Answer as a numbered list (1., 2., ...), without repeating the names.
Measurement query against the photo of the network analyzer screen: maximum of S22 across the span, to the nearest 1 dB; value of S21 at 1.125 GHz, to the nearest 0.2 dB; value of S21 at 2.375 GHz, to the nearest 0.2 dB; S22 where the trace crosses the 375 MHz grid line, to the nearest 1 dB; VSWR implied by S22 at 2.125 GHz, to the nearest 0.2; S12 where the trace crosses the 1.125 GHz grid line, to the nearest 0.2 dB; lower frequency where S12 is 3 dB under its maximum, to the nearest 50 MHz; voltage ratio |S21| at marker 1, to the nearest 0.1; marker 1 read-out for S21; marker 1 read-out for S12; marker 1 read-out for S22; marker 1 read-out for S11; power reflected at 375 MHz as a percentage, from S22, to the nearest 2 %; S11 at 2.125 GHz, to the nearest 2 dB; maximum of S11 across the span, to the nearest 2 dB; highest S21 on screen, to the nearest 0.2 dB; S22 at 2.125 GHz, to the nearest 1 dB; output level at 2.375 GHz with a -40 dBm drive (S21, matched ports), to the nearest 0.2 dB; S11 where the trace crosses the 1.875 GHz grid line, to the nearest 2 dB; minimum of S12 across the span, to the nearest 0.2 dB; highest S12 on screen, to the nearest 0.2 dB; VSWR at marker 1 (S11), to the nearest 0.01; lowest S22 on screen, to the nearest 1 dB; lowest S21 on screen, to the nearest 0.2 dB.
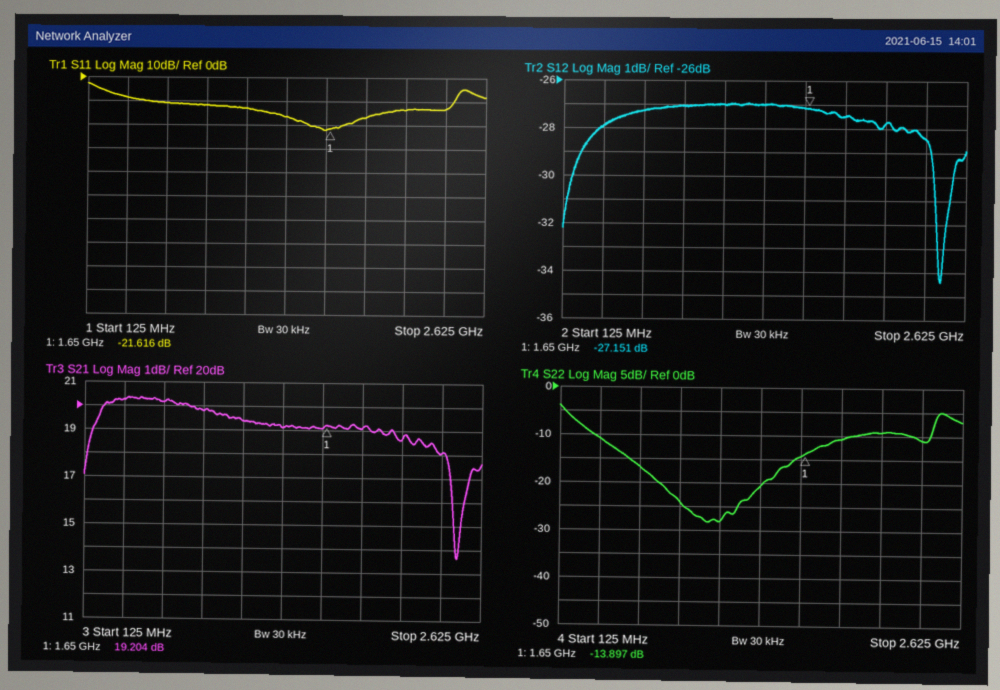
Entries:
1. -4 dB
2. 19.4 dB
3. 18.0 dB
4. -11 dB
5. 2.0
6. -27.0 dB
7. 200 MHz
8. 9.1
9. 19.204 dB
10. -27.151 dB
11. -13.897 dB
12. -21.616 dB
13. 8 %
14. -14 dB
15. -2 dB
16. 20.4 dB
17. -9 dB
18. -22.0 dBm
19. -16 dB
20. -34.4 dB
21. -27.0 dB
22. 1.18
23. -28 dB
24. 13.6 dB
